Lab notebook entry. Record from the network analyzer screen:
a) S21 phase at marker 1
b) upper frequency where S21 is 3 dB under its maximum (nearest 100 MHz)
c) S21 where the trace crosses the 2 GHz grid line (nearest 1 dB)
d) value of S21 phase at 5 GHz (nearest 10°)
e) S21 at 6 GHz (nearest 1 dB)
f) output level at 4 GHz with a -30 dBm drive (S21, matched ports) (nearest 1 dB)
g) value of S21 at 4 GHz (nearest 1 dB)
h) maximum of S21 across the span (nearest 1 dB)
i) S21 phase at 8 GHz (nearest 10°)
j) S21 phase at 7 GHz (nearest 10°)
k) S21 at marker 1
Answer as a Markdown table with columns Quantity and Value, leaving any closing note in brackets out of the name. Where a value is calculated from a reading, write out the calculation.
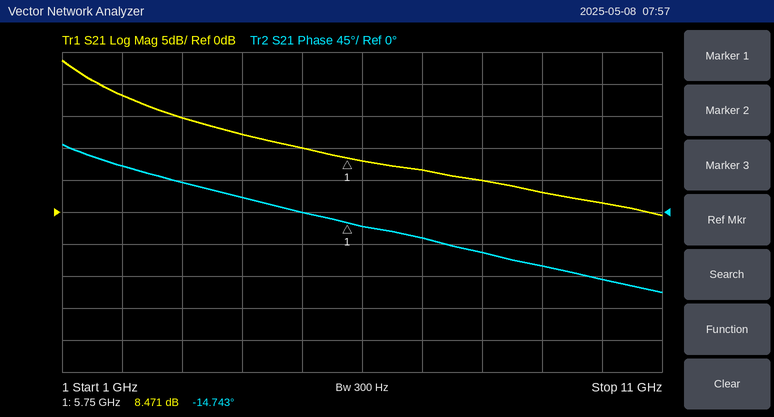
| Quantity | Value |
|---|---|
| S21 phase at marker 1 | -14.743° |
| upper frequency where S21 is 3 dB under its maximum | 1.5 GHz |
| S21 where the trace crosses the 2 GHz grid line | 18 dB |
| value of S21 phase at 5 GHz | 0° |
| S21 at 6 GHz | 8 dB |
| output level at 4 GHz with a -30 dBm drive (S21, matched ports) | -30 dBm + (12 dB) = -18 dBm |
| value of S21 at 4 GHz | 12 dB |
| maximum of S21 across the span | 24 dB |
| S21 phase at 8 GHz | -60° |
| S21 phase at 7 GHz | -40° |
| S21 at marker 1 | 8.471 dB |
